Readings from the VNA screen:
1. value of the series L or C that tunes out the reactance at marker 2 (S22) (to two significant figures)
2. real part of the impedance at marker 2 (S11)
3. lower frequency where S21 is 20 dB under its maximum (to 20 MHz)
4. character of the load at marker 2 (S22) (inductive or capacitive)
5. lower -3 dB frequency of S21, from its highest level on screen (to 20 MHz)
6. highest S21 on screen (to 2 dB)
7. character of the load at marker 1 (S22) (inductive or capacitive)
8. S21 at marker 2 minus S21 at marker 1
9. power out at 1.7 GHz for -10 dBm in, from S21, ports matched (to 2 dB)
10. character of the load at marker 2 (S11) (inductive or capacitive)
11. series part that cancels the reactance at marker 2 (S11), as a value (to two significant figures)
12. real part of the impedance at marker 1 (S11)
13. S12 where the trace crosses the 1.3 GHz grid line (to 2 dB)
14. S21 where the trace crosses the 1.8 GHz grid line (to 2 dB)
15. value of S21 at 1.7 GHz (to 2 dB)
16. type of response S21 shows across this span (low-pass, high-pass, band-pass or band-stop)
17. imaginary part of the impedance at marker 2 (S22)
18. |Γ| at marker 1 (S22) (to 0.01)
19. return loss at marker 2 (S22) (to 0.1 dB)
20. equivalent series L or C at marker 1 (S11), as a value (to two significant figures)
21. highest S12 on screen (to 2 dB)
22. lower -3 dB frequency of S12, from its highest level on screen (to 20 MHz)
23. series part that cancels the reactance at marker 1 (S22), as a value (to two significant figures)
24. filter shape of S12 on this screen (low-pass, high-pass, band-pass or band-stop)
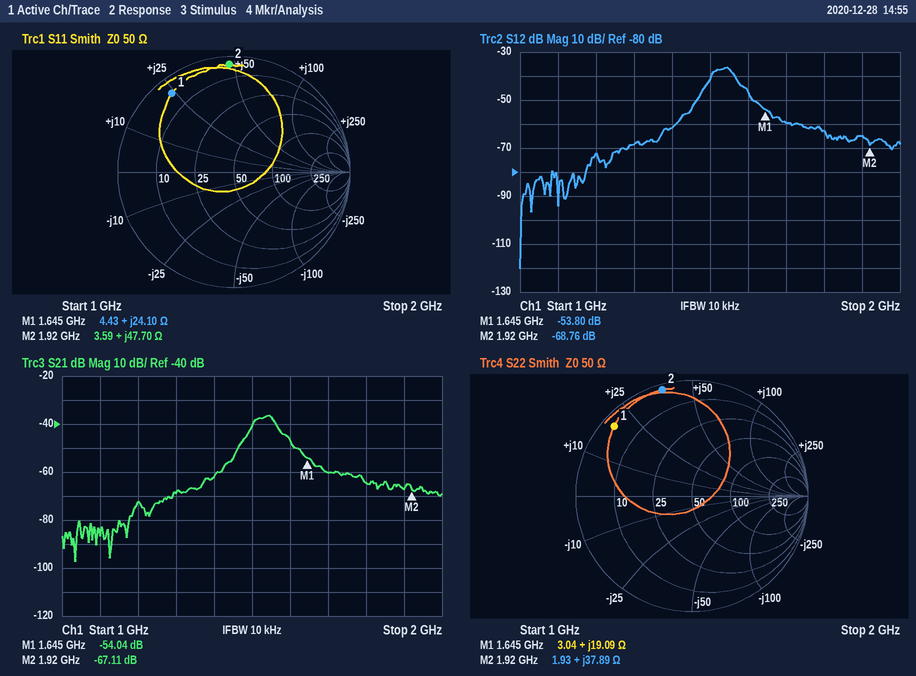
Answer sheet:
2.2 pF
3.59 Ω
1.44 GHz
inductive
1.50 GHz
-36 dB
inductive
-13.07 dB
-70 dBm
inductive
1.7 pF
4.43 Ω
-68 dB
-64 dB
-60 dB
band-pass
+37.89 Ω
0.90
0.4 dB
2.3 nH
-36 dB
1.50 GHz
5.1 pF
band-pass
